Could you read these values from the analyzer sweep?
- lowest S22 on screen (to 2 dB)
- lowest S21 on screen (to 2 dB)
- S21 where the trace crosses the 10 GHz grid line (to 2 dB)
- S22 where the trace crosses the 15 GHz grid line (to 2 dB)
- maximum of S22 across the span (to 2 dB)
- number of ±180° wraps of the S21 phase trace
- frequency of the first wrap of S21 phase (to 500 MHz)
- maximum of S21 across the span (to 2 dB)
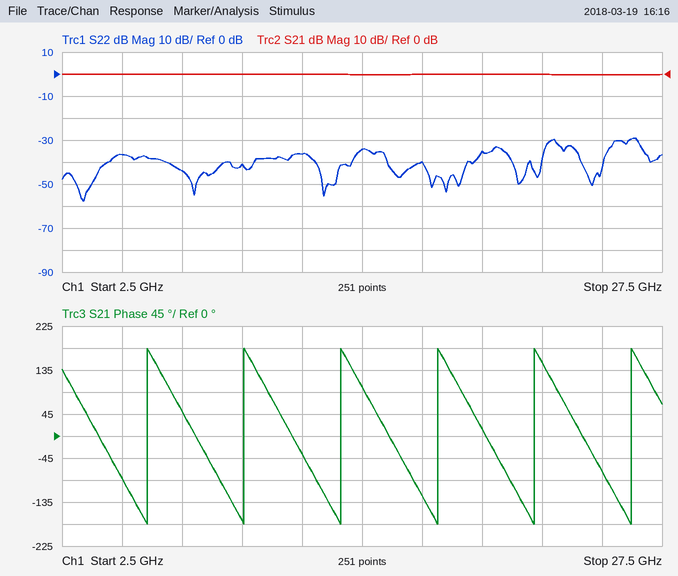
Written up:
-58 dB
0 dB
0 dB
-34 dB
-30 dB
6
6.0 GHz
0 dB
